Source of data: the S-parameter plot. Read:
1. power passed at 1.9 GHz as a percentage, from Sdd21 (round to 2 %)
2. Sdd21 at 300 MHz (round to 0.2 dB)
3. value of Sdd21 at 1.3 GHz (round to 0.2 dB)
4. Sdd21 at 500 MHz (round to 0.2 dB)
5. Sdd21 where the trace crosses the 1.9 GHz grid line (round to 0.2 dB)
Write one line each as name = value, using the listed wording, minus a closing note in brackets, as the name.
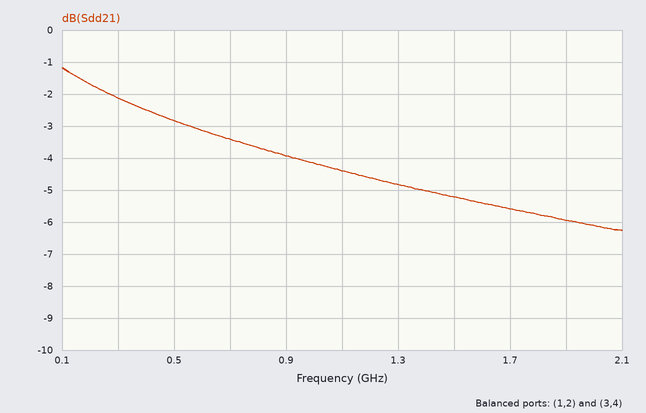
power passed at 1.9 GHz as a percentage, from Sdd21 = 26 %
Sdd21 at 300 MHz = -2.2 dB
value of Sdd21 at 1.3 GHz = -4.8 dB
Sdd21 at 500 MHz = -2.8 dB
Sdd21 where the trace crosses the 1.9 GHz grid line = -6.0 dB
